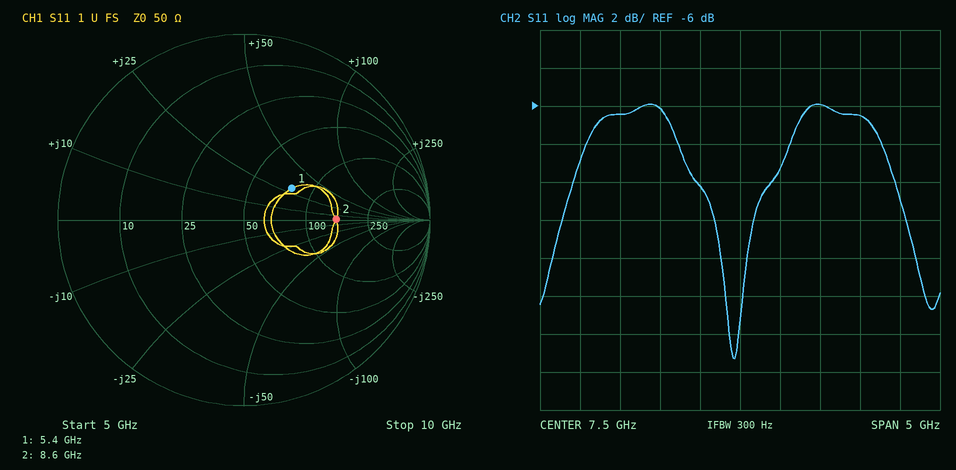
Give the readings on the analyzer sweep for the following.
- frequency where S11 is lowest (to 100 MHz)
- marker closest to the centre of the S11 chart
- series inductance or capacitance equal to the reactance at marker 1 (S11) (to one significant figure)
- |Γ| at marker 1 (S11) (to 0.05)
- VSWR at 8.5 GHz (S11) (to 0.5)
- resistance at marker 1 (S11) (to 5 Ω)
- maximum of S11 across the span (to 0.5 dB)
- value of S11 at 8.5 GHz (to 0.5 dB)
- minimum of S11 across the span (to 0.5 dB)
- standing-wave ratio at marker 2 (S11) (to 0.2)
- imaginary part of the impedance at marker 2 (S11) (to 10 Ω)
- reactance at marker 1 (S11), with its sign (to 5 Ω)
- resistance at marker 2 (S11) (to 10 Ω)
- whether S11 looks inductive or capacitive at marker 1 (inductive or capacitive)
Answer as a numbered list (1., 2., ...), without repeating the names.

1. 7.4 GHz
2. marker 1
3. 900 pH
4. 0.30
5. 3.0
6. 80 Ω
7. -6.0 dB
8. -6.0 dB
9. -19.5 dB
10. 3.0
11. 0 Ω
12. +30 Ω
13. 150 Ω
14. inductive
